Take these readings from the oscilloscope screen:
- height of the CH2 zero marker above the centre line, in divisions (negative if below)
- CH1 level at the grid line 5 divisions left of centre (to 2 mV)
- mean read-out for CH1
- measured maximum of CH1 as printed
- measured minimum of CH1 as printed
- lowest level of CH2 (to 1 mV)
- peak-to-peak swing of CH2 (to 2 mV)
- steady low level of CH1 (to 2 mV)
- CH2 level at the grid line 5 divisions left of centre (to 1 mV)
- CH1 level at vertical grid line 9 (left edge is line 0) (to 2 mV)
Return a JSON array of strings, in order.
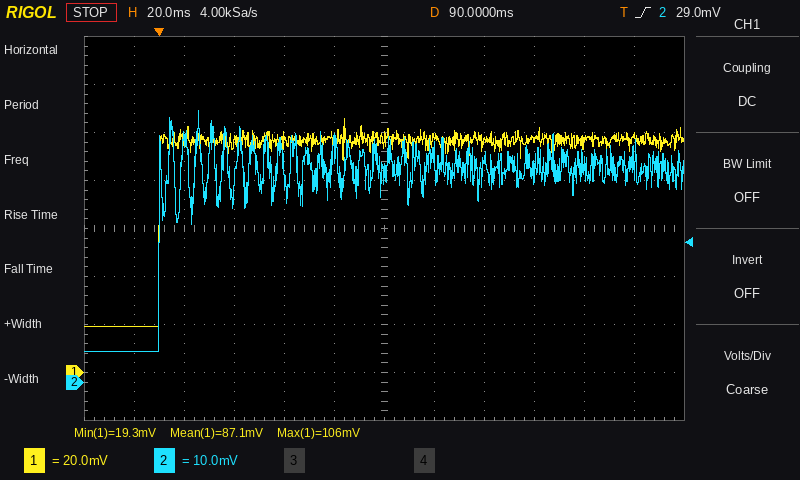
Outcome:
["-3.2 div", "20 mV", "87.1 mV", "106 mV", "19.3 mV", "6 mV", "50 mV", "20 mV", "6 mV", "98 mV"]
